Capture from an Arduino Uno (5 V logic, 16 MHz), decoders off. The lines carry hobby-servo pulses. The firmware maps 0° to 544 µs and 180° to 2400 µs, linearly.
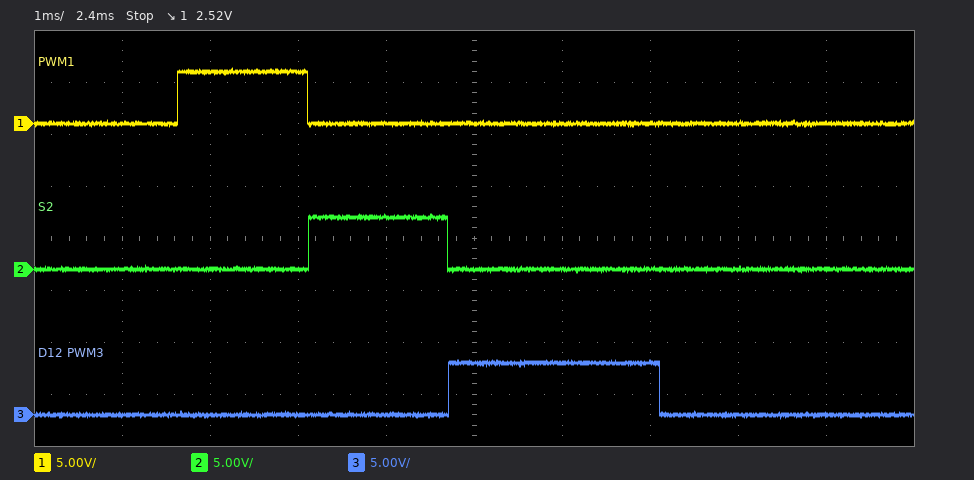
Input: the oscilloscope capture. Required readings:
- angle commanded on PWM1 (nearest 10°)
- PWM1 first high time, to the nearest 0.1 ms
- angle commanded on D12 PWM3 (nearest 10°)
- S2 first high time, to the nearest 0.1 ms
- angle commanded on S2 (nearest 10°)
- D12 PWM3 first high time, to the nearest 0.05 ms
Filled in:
90°
1.5 ms
180°
1.6 ms
100°
2.40 ms
